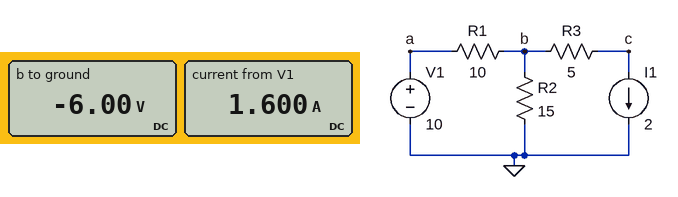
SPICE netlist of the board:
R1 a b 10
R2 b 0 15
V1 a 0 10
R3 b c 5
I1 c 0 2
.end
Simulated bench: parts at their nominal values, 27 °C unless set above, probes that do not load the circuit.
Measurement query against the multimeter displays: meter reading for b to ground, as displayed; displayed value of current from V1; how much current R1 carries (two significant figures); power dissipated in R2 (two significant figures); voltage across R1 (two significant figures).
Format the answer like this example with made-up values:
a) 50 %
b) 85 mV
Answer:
a) -6.00 V
b) 1.600 A
c) 1.6 A
d) 2.4 W
e) 16 V
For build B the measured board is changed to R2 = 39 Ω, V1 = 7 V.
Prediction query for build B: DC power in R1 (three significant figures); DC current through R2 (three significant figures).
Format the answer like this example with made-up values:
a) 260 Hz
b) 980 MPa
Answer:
a) 30.1 W
b) 265 mA
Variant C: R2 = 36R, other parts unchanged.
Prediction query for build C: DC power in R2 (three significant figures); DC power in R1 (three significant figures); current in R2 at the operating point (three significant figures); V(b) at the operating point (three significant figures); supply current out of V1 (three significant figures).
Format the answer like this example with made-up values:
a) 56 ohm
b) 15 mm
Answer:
a) 1.70 W
b) 31.8 W
c) 217 mA
d) -7.83 V
e) 1.78 A
